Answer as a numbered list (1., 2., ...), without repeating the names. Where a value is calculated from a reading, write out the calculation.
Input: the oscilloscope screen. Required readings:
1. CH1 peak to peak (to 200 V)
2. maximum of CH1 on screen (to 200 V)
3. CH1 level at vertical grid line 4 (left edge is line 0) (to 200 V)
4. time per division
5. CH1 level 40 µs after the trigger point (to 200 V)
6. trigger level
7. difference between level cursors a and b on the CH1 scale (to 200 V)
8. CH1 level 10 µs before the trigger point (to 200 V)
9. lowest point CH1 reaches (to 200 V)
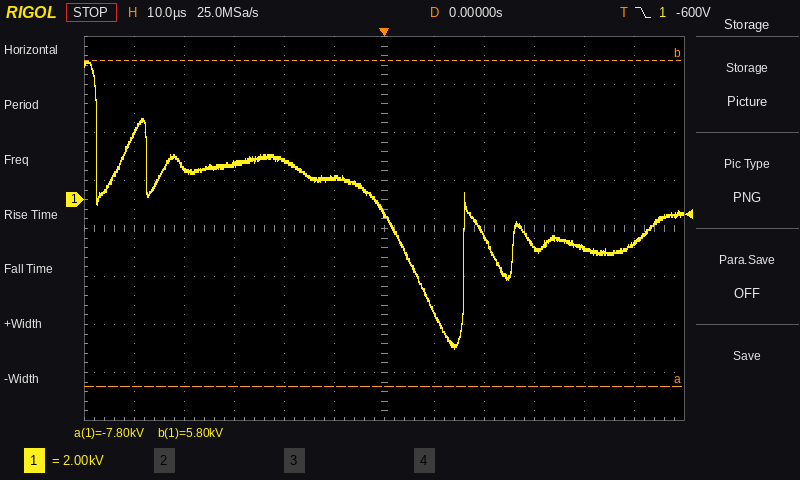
1. 5.8 kV − (-6.2 kV) = 12.0 kV
2. 5.8 kV
3. 1.6 kV
4. 10 µs
5. -2.0 kV
6. -600 V
7. 13.6 kV
8. 1.0 kV
9. -6.2 kV
